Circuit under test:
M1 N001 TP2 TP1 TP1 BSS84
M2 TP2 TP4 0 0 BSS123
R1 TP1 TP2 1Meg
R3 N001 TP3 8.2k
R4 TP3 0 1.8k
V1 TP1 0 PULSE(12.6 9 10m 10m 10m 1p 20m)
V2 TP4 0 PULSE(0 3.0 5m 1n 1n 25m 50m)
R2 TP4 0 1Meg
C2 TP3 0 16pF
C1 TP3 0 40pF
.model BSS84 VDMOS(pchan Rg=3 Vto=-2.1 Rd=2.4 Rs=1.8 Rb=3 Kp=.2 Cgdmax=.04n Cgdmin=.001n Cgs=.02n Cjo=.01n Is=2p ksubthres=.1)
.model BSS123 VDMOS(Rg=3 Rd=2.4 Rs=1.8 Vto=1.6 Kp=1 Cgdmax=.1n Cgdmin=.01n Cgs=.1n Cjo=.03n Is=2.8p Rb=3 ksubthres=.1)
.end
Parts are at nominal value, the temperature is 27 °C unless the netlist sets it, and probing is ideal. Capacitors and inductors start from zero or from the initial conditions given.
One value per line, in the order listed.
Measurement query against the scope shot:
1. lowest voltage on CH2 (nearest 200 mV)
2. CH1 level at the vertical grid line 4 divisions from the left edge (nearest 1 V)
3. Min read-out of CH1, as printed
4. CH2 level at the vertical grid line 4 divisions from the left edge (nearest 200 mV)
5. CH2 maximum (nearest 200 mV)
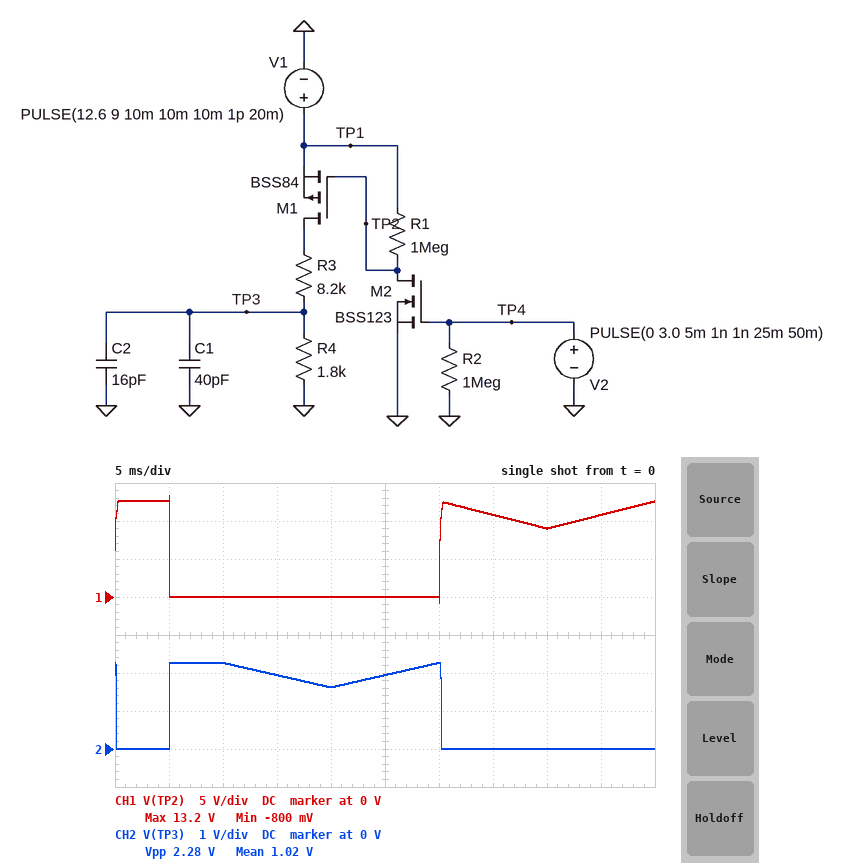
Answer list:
0 V
0 V
-800 mV
1.6 V
2.2 V
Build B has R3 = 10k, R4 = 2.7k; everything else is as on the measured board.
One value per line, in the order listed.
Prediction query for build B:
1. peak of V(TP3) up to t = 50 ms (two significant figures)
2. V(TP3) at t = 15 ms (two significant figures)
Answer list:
2.7 V
2.3 V
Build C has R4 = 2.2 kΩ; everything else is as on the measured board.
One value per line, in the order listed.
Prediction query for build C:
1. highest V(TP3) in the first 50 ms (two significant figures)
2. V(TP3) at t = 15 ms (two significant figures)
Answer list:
2.7 V
2.3 V
